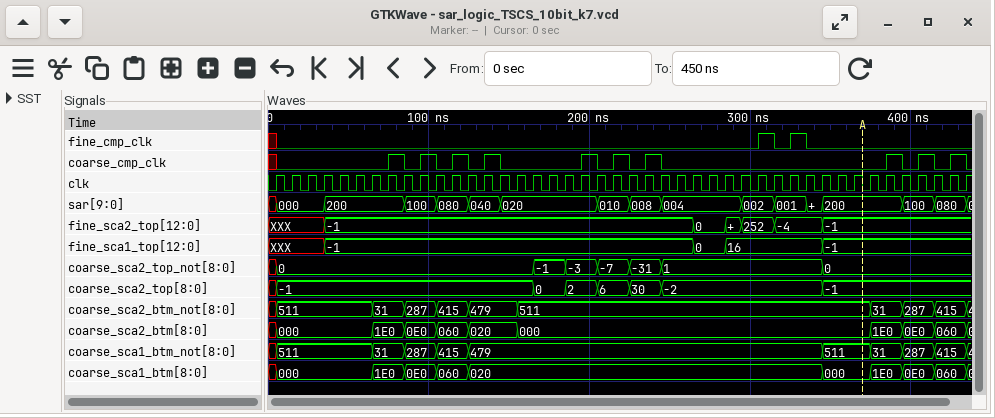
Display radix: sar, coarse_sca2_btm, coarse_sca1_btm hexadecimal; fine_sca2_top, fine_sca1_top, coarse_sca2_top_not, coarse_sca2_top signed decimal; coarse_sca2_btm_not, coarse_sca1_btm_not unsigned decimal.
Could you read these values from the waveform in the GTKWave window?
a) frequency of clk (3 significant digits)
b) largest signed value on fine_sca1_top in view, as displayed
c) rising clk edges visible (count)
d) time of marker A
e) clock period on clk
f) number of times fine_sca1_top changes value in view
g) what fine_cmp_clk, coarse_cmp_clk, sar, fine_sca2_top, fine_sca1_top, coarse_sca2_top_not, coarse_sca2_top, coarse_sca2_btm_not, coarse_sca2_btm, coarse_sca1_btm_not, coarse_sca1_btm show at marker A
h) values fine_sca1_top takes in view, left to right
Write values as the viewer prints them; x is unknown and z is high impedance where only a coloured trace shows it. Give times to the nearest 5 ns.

100 MHz
16
44
370 ns
10 ns
4
fine_cmp_clk=0, coarse_cmp_clk=0, sar=200, fine_sca2_top=-1, fine_sca1_top=-1, coarse_sca2_top_not=0, coarse_sca2_top=-1, coarse_sca2_btm_not=511, coarse_sca2_btm=000, coarse_sca1_btm_not=511, coarse_sca1_btm=000
XXX, -1, 0, 16, -1
